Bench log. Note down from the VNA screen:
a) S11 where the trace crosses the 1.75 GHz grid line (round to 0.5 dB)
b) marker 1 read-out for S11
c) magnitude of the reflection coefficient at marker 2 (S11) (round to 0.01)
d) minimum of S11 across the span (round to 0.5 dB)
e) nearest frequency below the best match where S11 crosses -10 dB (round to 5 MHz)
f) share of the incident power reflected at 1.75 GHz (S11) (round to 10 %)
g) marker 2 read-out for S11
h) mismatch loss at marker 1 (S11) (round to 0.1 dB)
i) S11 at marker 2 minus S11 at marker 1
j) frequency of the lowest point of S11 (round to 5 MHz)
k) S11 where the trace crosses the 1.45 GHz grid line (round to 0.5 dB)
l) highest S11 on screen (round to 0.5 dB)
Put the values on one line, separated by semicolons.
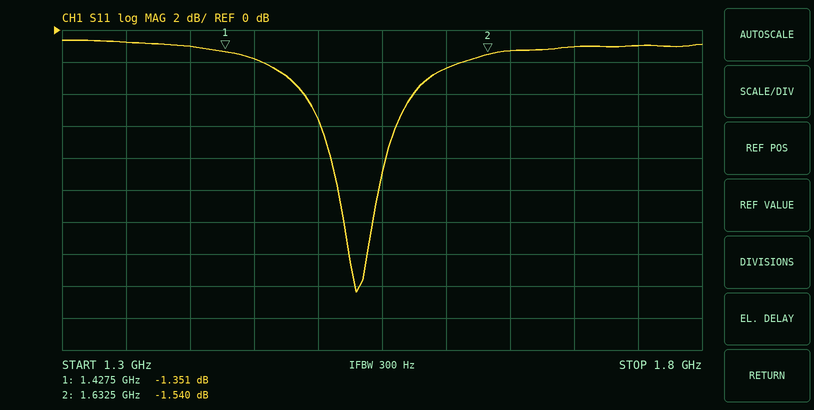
-1.0 dB; -1.351 dB; 0.84; -16.5 dB; 1.515 GHz; 80 %; -1.540 dB; 5.7 dB; -0.189 dB; 1.530 GHz; -2.0 dB; -0.5 dB
